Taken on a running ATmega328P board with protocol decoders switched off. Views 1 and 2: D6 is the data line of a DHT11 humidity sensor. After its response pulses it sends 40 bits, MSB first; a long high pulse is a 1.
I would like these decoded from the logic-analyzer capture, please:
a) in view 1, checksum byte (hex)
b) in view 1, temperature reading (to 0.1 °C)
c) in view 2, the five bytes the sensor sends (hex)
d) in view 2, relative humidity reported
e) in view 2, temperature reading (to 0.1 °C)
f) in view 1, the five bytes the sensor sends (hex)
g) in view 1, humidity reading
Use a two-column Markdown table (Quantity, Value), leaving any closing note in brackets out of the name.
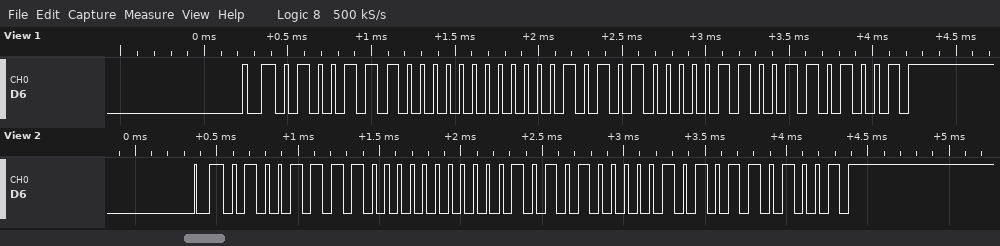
| Quantity | Value |
|---|---|
| in view 1, checksum byte | 0x69 |
| in view 1, temperature reading | 21.6 °C |
| in view 2, the five bytes the sensor sends | 4F 00 15 05 69 |
| in view 2, relative humidity reported | 79 % |
| in view 2, temperature reading | 21.5 °C |
| in view 1, the five bytes the sensor sends | 4E 00 15 06 69 |
| in view 1, humidity reading | 78 % |
